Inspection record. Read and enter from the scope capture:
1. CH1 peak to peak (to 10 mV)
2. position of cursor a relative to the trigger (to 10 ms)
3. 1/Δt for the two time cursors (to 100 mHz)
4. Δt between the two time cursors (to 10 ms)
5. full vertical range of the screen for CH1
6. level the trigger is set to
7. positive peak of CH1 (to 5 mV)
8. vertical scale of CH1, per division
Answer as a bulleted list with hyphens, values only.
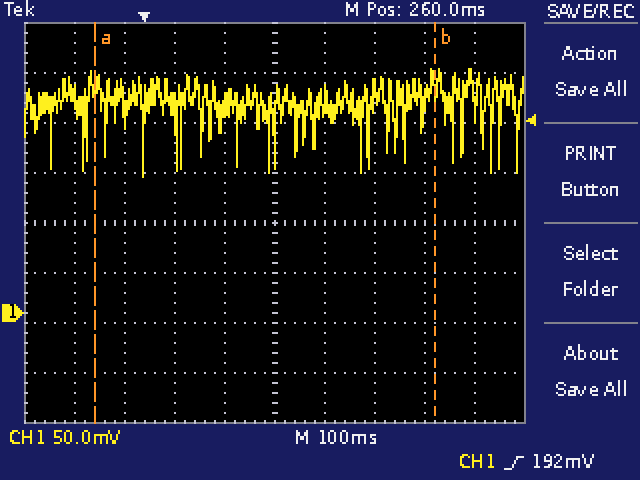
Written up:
- 110 mV
- -100 ms
- 1.5 Hz
- 680 ms
- 400 mV
- 192 mV
- 245 mV
- 50 mV
